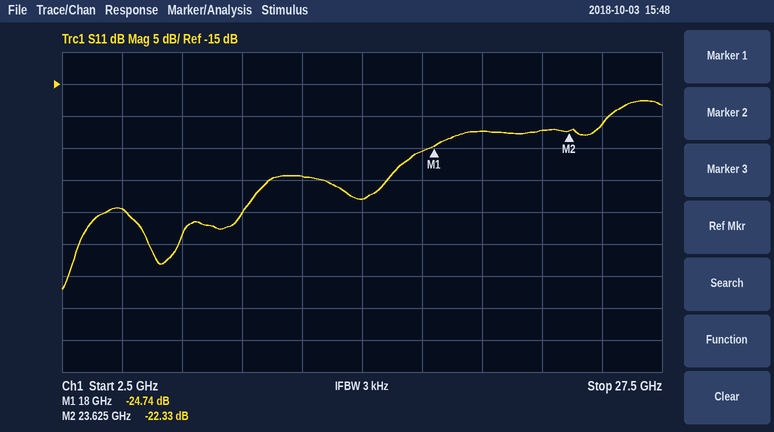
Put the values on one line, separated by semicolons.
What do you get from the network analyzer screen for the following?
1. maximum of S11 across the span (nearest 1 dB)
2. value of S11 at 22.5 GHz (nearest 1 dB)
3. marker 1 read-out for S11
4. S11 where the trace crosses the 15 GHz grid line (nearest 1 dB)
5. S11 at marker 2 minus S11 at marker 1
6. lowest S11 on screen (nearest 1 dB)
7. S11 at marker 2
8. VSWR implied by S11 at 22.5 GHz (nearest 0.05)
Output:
-18 dB; -22 dB; -24.74 dB; -33 dB; 2.41 dB; -47 dB; -22.33 dB; 1.15
